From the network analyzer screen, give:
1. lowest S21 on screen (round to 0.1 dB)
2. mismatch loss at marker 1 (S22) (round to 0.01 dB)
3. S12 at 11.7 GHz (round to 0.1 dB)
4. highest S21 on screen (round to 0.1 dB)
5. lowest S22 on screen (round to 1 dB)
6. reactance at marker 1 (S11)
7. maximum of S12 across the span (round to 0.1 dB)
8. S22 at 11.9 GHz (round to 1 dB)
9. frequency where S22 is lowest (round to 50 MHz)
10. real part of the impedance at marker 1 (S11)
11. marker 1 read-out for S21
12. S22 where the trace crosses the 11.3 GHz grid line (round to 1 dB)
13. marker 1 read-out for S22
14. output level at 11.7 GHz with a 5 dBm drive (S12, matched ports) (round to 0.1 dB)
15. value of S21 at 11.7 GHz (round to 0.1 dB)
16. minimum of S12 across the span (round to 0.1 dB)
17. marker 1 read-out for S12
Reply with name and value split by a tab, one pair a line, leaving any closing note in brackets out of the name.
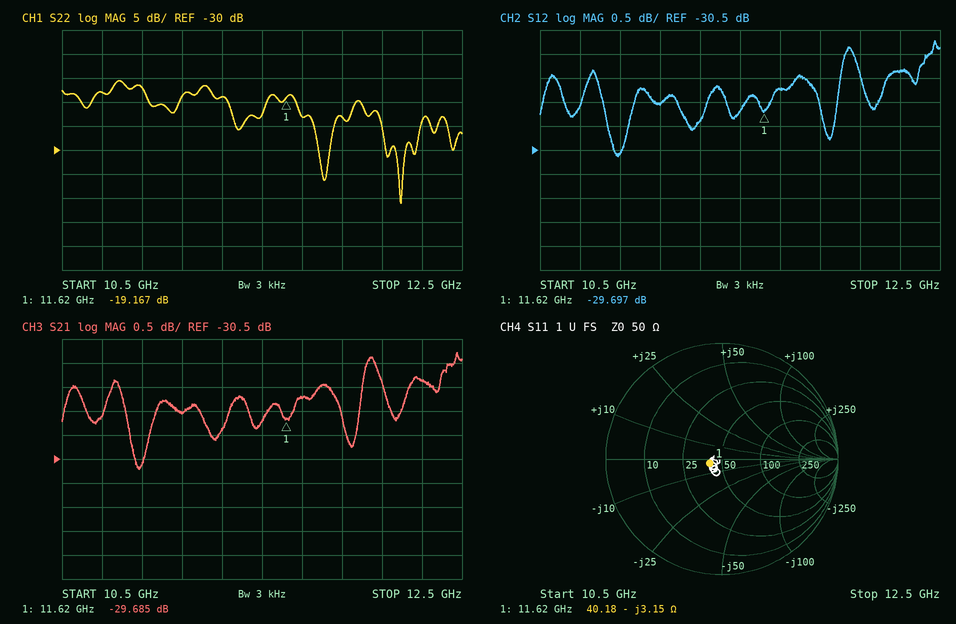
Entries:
lowest S21 on screen	-30.7 dB
mismatch loss at marker 1 (S22)	0.05 dB
S12 at 11.7 GHz	-29.2 dB
highest S21 on screen	-28.3 dB
lowest S22 on screen	-41 dB
reactance at marker 1	-3.15 Ω
maximum of S12 across the span	-28.2 dB
S22 at 11.9 GHz	-23 dB
frequency where S22 is lowest	12.20 GHz
real part of the impedance at marker 1	40.18 Ω
marker 1 read-out for S21	-29.685 dB
S22 where the trace crosses the 11.3 GHz grid line	-19 dB
marker 1 read-out for S22	-19.167 dB
output level at 11.7 GHz with a 5 dBm drive (S12, matched ports)	-24.2 dBm
value of S21 at 11.7 GHz	-29.2 dB
minimum of S12 across the span	-30.6 dB
marker 1 read-out for S12	-29.697 dB
